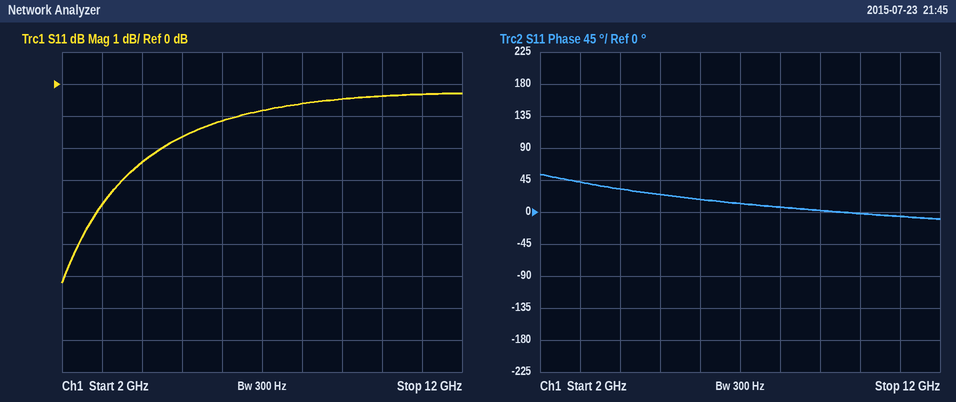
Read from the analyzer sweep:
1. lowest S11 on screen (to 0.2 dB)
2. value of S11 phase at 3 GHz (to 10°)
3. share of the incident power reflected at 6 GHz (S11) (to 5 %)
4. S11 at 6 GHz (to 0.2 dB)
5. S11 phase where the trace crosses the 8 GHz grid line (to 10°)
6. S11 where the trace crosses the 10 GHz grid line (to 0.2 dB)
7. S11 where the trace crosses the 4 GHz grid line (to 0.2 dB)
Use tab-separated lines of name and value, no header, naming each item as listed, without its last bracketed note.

lowest S11 on screen	-6.2 dB
value of S11 phase at 3 GHz	40°
share of the incident power reflected at 6 GHz (S11)	75 %
S11 at 6 GHz	-1.2 dB
S11 phase where the trace crosses the 8 GHz grid line	10°
S11 where the trace crosses the 10 GHz grid line	-0.4 dB
S11 where the trace crosses the 4 GHz grid line	-2.4 dB
